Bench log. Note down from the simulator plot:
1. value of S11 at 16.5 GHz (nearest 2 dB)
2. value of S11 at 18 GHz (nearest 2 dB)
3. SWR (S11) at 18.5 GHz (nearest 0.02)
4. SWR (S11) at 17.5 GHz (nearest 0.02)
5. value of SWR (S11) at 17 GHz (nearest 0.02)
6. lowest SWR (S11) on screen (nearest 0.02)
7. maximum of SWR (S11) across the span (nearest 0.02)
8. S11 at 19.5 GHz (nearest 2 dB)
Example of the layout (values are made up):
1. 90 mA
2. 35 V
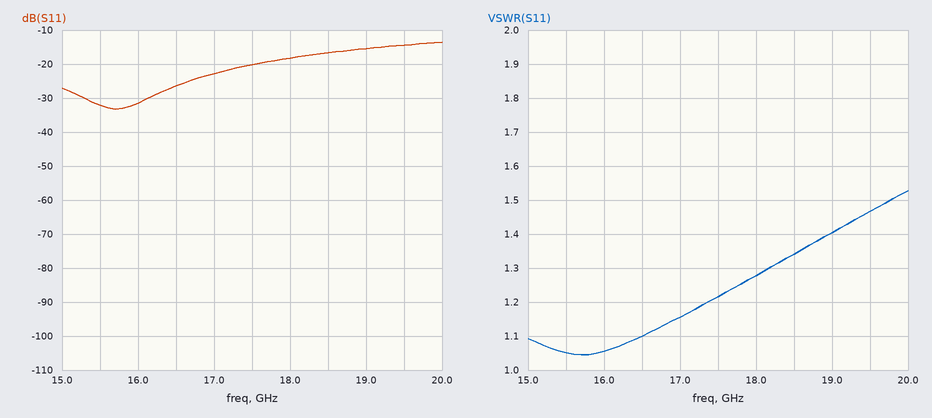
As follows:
1. -26 dB
2. -18 dB
3. 1.34
4. 1.22
5. 1.16
6. 1.04
7. 1.52
8. -14 dB
